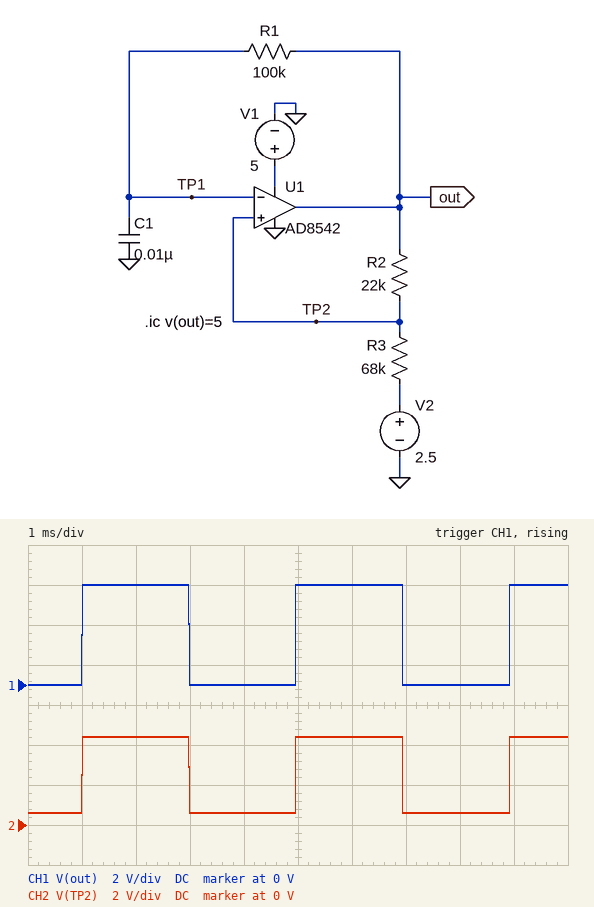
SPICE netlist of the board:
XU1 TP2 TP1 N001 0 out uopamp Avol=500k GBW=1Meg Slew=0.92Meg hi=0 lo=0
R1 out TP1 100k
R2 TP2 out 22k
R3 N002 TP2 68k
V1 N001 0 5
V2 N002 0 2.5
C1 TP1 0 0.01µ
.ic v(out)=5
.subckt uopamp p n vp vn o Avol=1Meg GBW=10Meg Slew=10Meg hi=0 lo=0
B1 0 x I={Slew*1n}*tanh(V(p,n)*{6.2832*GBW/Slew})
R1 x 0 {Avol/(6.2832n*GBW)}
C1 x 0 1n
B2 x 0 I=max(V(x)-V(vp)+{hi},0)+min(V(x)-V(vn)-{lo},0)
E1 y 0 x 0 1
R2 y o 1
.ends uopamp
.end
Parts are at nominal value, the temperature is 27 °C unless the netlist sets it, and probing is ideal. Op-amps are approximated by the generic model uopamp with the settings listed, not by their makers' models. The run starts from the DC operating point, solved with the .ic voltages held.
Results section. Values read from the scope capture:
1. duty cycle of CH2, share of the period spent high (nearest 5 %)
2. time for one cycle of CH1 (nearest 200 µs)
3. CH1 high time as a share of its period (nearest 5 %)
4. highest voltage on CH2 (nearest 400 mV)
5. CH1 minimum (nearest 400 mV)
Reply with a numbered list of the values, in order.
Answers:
1. 50 %
2. 4.0 ms
3. 50 %
4. 4.4 V
5. 0 V
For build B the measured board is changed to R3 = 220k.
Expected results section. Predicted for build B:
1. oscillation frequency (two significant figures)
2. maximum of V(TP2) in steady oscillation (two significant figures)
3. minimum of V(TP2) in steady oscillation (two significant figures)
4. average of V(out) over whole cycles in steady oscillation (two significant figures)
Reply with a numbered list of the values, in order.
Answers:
1. 160 Hz
2. 4.8 V
3. 230 mV
4. 2.5 V
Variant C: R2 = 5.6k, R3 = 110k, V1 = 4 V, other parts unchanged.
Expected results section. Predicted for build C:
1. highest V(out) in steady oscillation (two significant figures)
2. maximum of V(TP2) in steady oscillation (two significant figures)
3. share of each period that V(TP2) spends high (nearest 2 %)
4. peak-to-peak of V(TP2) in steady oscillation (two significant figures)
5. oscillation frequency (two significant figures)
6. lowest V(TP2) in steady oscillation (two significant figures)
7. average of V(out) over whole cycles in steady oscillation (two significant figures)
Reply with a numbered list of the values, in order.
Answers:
1. 4.0 V
2. 3.9 V
3. 54 %
4. 3.8 V
5. 130 Hz
6. 120 mV
7. 2.1 V
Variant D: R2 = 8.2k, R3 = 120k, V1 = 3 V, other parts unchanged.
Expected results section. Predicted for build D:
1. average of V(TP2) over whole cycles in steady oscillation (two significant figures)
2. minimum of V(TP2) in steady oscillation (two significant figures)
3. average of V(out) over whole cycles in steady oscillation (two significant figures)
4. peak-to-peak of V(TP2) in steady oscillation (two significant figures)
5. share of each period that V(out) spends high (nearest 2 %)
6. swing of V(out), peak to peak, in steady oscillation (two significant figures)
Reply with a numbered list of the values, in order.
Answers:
1. 1.9 V
2. 160 mV
3. 1.8 V
4. 2.8 V
5. 60 %
6. 3.0 V
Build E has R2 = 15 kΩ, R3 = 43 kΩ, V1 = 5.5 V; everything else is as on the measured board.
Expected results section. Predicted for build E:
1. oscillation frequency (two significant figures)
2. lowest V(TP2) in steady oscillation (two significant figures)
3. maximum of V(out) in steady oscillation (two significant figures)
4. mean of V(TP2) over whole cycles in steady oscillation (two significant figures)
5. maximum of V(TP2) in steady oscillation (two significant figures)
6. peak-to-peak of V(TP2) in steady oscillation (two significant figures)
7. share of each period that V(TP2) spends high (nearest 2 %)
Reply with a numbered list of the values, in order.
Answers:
1. 260 Hz
2. 650 mV
3. 5.5 V
4. 2.6 V
5. 4.7 V
6. 4.1 V
7. 48 %
